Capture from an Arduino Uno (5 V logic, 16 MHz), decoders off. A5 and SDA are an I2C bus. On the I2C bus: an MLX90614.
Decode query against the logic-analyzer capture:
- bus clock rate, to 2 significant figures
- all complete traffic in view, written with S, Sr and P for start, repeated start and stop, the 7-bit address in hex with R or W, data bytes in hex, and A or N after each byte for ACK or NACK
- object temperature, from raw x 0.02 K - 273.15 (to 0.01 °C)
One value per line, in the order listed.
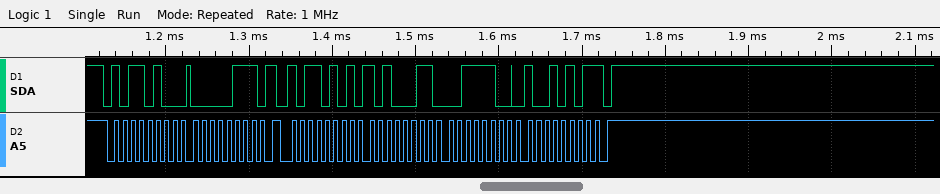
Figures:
100 kHz
S 5AW A 07 A Sr 5AR A A3 A 3C A 95 N P
37.31 °C
